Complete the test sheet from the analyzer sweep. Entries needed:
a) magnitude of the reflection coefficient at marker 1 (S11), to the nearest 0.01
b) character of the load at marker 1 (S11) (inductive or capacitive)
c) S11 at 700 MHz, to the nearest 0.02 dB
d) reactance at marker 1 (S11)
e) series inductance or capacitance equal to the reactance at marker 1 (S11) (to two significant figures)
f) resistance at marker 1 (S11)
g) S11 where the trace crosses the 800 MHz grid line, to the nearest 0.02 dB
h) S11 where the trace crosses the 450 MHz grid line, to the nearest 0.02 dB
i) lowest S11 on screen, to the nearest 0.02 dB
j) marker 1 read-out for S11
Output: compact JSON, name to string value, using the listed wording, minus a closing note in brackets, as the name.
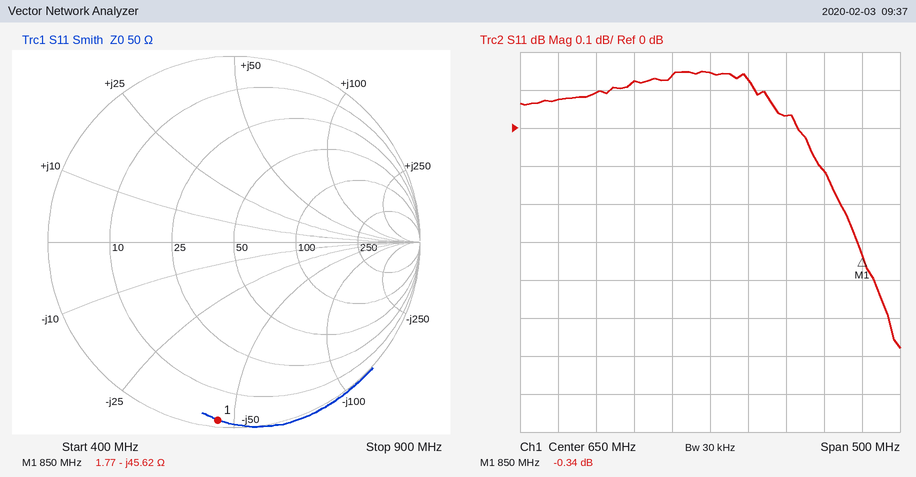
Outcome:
{"magnitude of the reflection coefficient at marker 1 (S11), to the nearest 0.01": "0.96", "character of the load at marker 1 (S11)": "capacitive", "S11 at 700 MHz, to the nearest 0.02 dB": "0.12 dB", "reactance at marker 1": "-45.62 Ω", "series inductance or capacitance equal to the reactance at marker 1 (S11)": "4.1 pF", "resistance at marker 1": "1.77 Ω", "S11 where the trace crosses the 800 MHz grid line, to the nearest 0.02 dB": "-0.12 dB", "S11 where the trace crosses the 450 MHz grid line, to the nearest 0.02 dB": "0.08 dB", "lowest S11 on screen, to the nearest 0.02 dB": "-0.58 dB", "marker 1 read-out for S11": "-0.34 dB"}
